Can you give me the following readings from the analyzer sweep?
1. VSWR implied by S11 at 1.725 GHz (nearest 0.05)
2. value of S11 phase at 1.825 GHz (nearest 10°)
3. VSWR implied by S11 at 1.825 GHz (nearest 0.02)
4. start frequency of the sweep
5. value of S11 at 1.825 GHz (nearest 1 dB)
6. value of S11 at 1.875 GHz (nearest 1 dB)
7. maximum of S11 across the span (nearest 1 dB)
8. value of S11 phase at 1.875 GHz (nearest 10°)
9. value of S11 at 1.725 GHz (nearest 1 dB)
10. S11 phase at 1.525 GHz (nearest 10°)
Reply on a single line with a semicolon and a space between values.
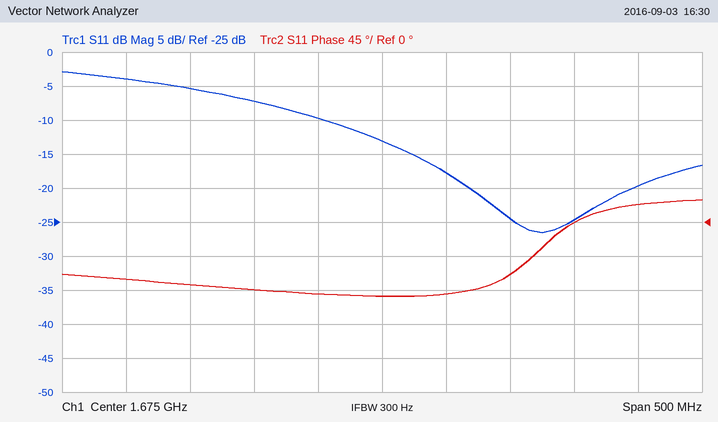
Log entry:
1.30; 0°; 1.12; 1.425 GHz; -25 dB; -20 dB; -3 dB; 20°; -18 dB; -80°
